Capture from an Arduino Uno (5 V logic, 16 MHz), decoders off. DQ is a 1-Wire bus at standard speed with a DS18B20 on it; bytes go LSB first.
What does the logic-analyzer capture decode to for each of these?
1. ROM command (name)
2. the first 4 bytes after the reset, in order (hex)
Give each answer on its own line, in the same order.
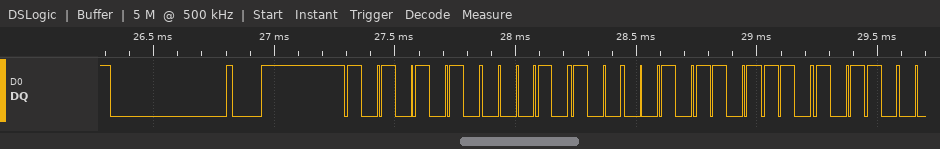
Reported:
Match ROM
55 28 B4 6B
